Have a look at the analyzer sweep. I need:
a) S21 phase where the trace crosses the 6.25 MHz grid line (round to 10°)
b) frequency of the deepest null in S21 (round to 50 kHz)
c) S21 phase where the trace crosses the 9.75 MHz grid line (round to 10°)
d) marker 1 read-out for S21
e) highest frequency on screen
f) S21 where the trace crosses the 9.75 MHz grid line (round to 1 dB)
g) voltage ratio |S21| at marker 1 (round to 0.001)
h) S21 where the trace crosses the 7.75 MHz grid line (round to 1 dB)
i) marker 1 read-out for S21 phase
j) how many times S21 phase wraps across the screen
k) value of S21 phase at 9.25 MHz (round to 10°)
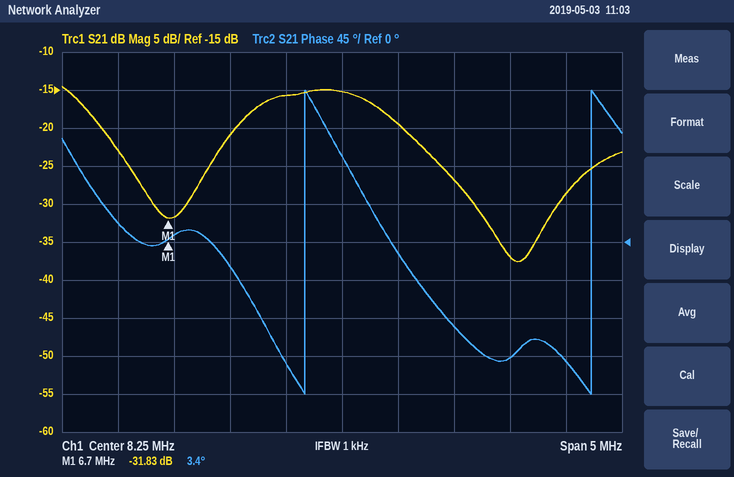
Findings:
20°
9.80 MHz
-140°
-31.83 dB
10.75 MHz
-37 dB
0.026
-16 dB
3.4°
2
-100°
